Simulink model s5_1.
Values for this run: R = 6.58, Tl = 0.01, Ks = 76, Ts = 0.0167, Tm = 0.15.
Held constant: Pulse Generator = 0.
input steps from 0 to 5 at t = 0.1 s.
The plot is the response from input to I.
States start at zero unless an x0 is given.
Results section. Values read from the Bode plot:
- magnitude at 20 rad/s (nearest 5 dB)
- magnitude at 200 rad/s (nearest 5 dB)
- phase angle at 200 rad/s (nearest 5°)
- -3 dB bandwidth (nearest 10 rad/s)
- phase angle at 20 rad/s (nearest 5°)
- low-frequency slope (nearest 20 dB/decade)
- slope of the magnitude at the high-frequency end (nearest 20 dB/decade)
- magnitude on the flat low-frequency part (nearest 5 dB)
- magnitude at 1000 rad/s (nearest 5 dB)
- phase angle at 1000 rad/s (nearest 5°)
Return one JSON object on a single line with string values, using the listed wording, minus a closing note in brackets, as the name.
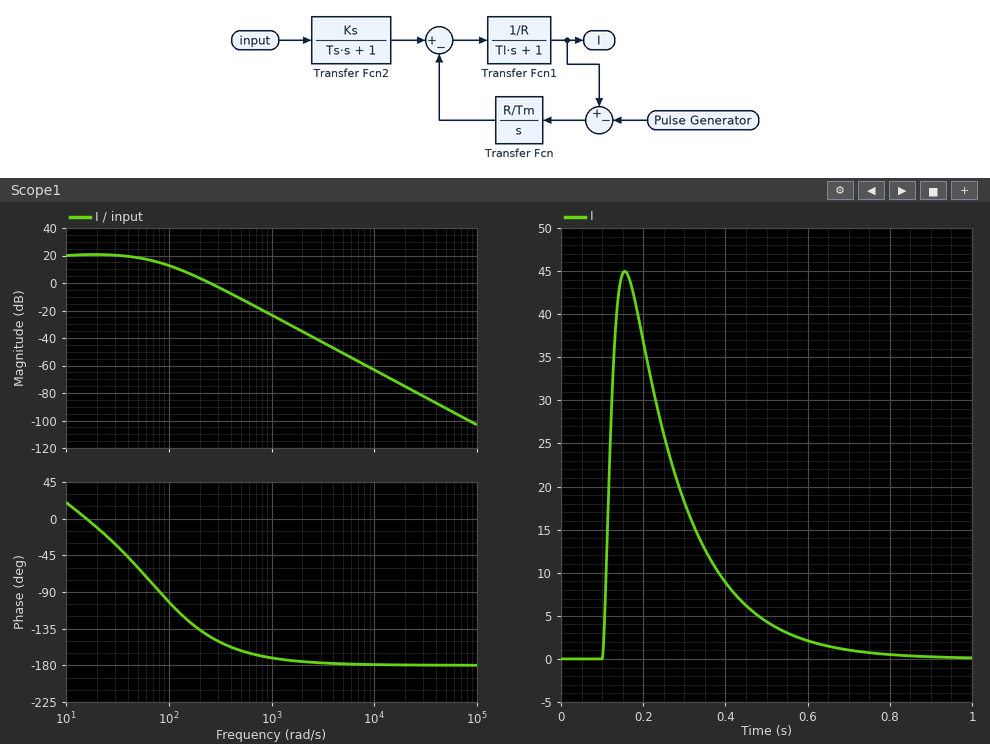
{"magnitude at 20 rad/s": "20 dB", "magnitude at 200 rad/s": "5 dB", "phase angle at 200 rad/s": "-135°", "-3 dB bandwidth": "60 rad/s", "phase angle at 20 rad/s": "-10°", "low-frequency slope": "0 dB/decade", "slope of the magnitude at the high-frequency end": "-40 dB/decade", "magnitude on the flat low-frequency part": "20 dB", "magnitude at 1000 rad/s": "-25 dB", "phase angle at 1000 rad/s": "-170°"}
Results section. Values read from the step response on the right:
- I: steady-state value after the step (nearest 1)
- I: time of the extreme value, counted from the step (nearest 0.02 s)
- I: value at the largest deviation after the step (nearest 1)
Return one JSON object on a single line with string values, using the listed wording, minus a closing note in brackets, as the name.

{"I: steady-state value after the step": "0", "I: time of the extreme value, counted from the step": "0.06 s", "I: value at the largest deviation after the step": "45"}
